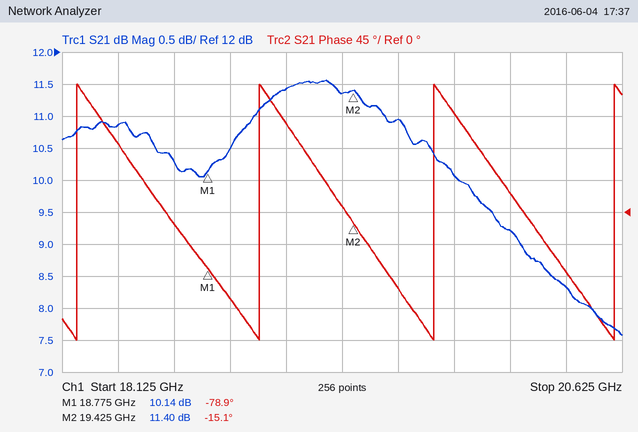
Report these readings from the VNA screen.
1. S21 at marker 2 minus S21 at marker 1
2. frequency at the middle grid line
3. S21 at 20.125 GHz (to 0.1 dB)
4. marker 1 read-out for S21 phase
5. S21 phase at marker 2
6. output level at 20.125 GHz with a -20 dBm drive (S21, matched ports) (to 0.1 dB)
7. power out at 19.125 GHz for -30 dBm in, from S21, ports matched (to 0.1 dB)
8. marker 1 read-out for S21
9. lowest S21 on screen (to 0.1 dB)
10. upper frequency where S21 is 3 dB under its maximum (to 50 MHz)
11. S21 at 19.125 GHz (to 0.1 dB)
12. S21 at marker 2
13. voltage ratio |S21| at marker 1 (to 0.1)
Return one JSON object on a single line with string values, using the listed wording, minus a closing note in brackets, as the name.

{"S21 at marker 2 minus S21 at marker 1": "1.26 dB", "frequency at the middle grid line": "19.375 GHz", "S21 at 20.125 GHz": "9.2 dB", "marker 1 read-out for S21 phase": "-78.9°", "S21 phase at marker 2": "-15.1°", "output level at 20.125 GHz with a -20 dBm drive (S21, matched ports)": "-10.8 dBm", "power out at 19.125 GHz for -30 dBm in, from S21, ports matched": "-18.6 dBm", "marker 1 read-out for S21": "10.14 dB", "lowest S21 on screen": "7.6 dB", "upper frequency where S21 is 3 dB under its maximum": "20.30 GHz", "S21 at 19.125 GHz": "11.4 dB", "S21 at marker 2": "11.40 dB", "voltage ratio |S21| at marker 1": "3.2"}
